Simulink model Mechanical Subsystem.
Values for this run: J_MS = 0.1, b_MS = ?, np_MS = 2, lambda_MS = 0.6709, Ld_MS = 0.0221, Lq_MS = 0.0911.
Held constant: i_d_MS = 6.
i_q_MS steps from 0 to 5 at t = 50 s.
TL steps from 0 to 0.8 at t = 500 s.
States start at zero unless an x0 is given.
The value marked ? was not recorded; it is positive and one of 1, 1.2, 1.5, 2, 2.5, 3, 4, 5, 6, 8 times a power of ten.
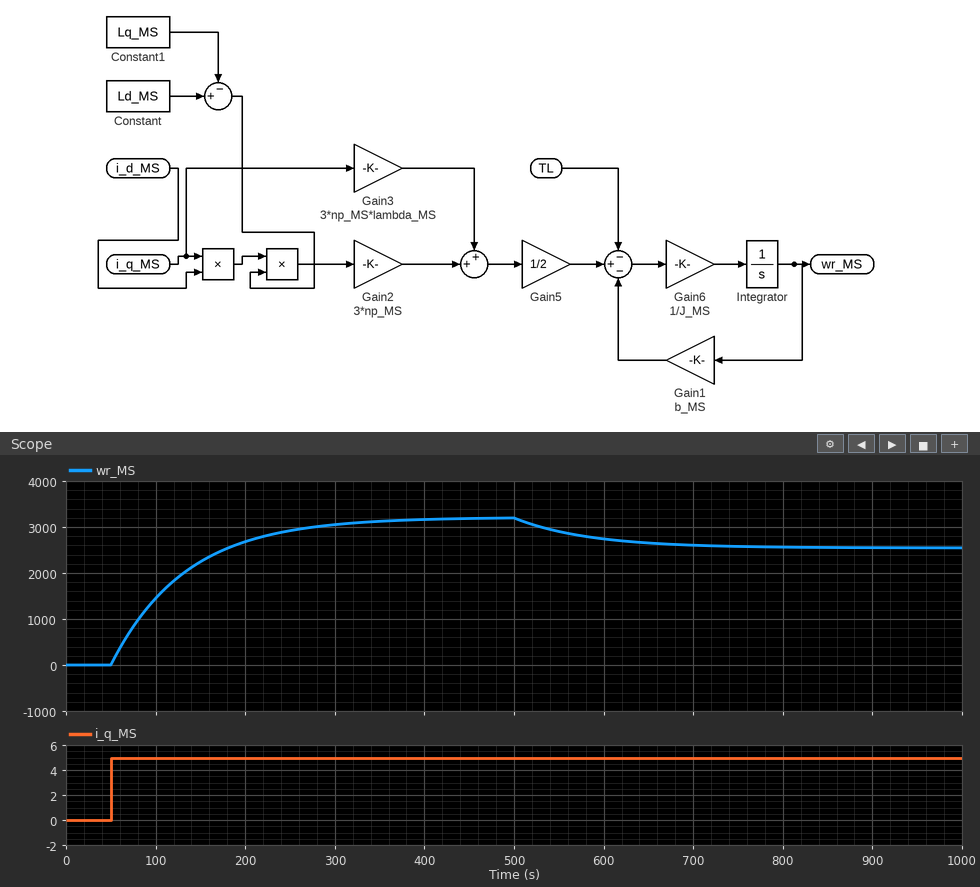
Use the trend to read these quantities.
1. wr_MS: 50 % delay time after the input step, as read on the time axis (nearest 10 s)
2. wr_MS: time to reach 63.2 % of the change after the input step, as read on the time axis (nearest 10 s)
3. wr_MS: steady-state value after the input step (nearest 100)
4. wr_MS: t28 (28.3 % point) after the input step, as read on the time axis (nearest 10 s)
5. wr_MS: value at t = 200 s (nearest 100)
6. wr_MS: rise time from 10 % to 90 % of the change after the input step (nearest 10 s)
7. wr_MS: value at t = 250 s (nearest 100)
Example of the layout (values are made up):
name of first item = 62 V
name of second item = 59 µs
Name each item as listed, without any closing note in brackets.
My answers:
wr_MS: 50 % delay time after the input step, as read on the time axis = 110 s
wr_MS: time to reach 63.2 % of the change after the input step, as read on the time axis = 130 s
wr_MS: steady-state value after the input step = 3200
wr_MS: t28 (28.3 % point) after the input step, as read on the time axis = 80 s
wr_MS: value at t = 200 s = 2700
wr_MS: rise time from 10 % to 90 % of the change after the input step = 180 s
wr_MS: value at t = 250 s = 2900
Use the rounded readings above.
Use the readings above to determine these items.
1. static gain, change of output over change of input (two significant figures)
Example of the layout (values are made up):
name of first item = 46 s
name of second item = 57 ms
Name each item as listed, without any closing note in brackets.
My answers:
static gain, change of output over change of input = 640
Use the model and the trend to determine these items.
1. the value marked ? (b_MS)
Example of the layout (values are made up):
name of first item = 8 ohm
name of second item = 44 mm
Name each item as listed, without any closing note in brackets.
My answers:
the value marked ? = 0.0012
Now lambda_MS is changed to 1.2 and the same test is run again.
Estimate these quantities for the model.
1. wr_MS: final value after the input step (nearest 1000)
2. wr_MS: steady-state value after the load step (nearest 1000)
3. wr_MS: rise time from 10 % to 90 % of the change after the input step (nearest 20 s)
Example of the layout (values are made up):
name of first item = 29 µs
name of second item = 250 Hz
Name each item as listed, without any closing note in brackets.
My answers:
wr_MS: final value after the input step = 10000
wr_MS: steady-state value after the load step = 9000
wr_MS: rise time from 10 % to 90 % of the change after the input step = 180 s
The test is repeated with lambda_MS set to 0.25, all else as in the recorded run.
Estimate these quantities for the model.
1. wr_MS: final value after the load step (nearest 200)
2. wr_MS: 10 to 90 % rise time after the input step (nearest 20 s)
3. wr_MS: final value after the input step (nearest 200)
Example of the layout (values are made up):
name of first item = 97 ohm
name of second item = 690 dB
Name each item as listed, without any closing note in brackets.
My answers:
wr_MS: final value after the load step = -2800
wr_MS: 10 to 90 % rise time after the input step = 180 s
wr_MS: final value after the input step = -2000
